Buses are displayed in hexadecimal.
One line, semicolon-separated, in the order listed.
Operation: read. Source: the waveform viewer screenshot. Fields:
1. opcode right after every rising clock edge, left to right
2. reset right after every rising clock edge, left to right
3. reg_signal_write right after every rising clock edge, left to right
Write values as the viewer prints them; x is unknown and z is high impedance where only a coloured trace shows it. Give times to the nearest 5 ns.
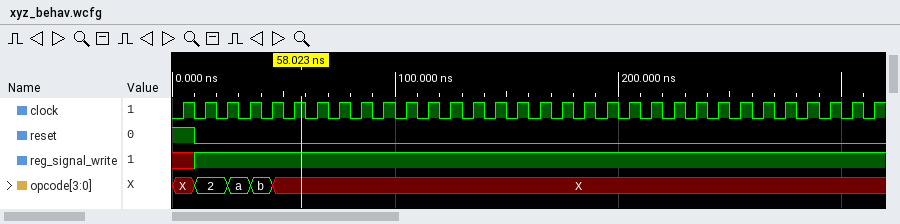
X, 2, a, b, X, X, X, X, X, X, X, X, X, X, X, X, X, X, X, X, X, X, X, X, X, X, X, X, X, X, X, X; 1 0 0 0 0 0 0 0 0 0 0 0 0 0 0 0 0 0 0 0 0 0 0 0 0 0 0 0 0 0 0 0; x 1 1 1 1 1 1 1 1 1 1 1 1 1 1 1 1 1 1 1 1 1 1 1 1 1 1 1 1 1 1 1
